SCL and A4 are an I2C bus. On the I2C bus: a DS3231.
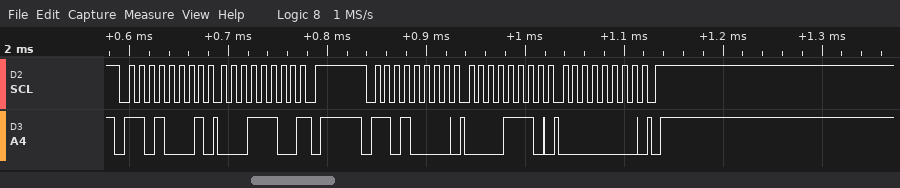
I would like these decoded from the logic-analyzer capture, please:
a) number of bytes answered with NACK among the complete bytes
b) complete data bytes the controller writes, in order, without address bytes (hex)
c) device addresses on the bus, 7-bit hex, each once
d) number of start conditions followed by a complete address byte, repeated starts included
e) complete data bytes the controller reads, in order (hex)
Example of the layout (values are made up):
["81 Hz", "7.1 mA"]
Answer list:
["1", "0E 00", "0x68", "2", "1C"]
